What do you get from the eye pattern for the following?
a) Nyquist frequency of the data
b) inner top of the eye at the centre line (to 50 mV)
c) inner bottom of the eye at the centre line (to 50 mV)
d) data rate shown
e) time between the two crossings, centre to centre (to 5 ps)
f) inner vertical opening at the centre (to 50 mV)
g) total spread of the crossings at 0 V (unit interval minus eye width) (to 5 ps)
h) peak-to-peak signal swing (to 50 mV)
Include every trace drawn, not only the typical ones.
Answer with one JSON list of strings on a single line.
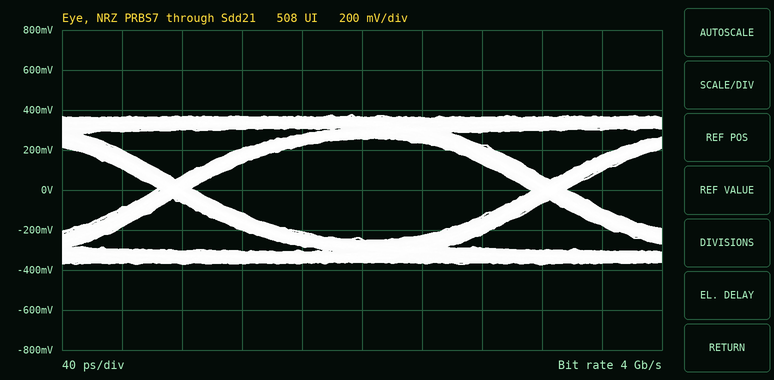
["2 GHz", "250 mV", "-250 mV", "4 Gb/s", "250 ps", "500 mV", "25 ps", "750 mV"]
